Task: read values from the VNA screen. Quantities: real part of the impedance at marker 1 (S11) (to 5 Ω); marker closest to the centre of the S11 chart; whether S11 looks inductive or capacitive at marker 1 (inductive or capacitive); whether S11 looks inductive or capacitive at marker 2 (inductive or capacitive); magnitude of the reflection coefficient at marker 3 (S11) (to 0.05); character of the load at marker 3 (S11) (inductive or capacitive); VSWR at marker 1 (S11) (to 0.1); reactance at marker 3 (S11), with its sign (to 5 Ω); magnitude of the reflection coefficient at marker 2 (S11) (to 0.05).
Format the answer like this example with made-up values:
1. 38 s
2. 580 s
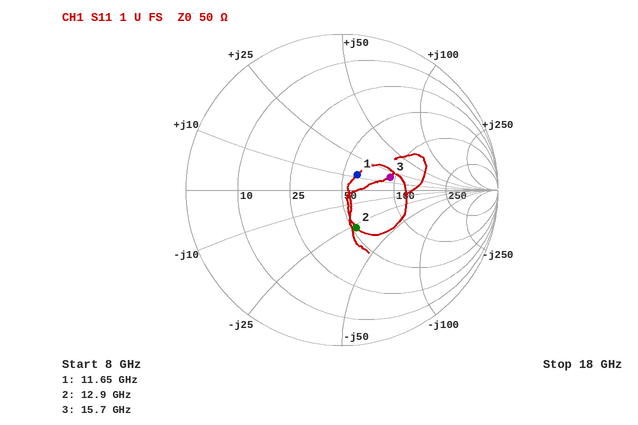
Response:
1. 60 Ω
2. marker 1
3. inductive
4. capacitive
5. 0.30
6. inductive
7. 1.3
8. +15 Ω
9. 0.25
